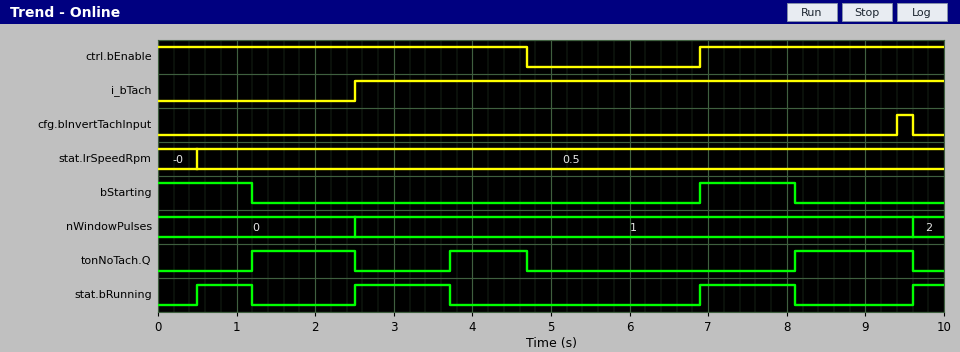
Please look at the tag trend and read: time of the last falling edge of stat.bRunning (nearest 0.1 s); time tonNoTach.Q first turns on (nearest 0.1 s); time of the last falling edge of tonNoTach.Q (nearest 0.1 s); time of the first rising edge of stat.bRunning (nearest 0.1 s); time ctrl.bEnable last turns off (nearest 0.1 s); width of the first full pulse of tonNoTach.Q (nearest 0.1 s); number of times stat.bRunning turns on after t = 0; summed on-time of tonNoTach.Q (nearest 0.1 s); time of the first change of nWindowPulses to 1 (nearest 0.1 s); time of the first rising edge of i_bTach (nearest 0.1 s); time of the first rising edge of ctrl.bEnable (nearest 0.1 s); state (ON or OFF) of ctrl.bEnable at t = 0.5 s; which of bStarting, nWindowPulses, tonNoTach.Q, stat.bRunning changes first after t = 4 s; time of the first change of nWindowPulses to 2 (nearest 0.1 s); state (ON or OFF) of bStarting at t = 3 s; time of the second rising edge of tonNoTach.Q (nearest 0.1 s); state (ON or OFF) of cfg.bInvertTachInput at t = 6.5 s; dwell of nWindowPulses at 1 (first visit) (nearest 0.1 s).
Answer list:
8.1 s
1.2 s
9.6 s
0.5 s
4.7 s
1.3 s
4
3.8 s
2.5 s
2.5 s
6.9 s
ON
tonNoTach.Q
9.6 s
OFF
3.7 s
OFF
7.1 s
